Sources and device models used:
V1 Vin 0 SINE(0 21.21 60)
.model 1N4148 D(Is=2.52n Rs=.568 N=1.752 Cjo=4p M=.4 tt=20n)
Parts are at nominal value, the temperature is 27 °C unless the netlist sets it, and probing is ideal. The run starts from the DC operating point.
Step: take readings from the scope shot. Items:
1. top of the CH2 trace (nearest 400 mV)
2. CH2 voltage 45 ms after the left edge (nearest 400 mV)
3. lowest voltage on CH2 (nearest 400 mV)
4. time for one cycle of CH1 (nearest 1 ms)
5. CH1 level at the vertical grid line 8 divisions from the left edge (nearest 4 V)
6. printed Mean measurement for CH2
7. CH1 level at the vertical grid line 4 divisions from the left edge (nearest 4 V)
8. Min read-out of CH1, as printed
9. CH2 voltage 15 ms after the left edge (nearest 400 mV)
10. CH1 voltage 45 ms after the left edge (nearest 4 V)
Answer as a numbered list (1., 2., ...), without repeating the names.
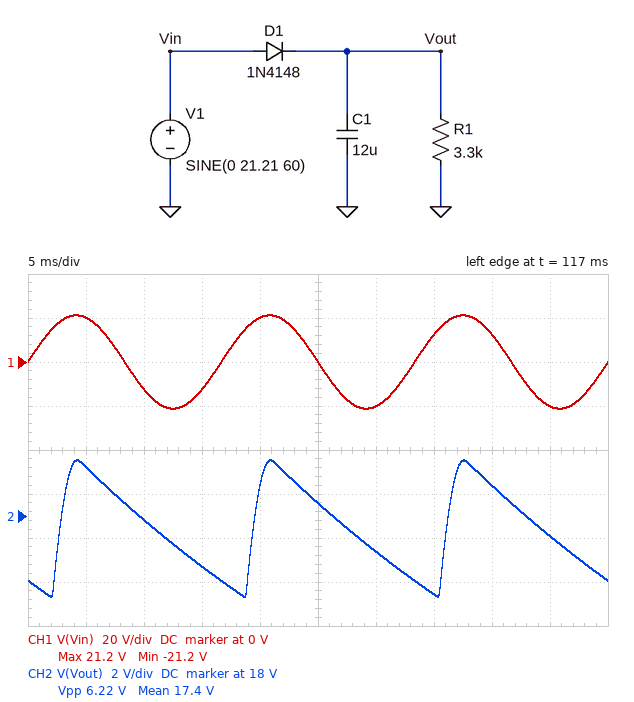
1. 20.4 V
2. 17.2 V
3. 14.4 V
4. 17 ms
5. 12 V
6. 17.4 V
7. 20 V
8. -21.2 V
9. 15.6 V
10. -20 V
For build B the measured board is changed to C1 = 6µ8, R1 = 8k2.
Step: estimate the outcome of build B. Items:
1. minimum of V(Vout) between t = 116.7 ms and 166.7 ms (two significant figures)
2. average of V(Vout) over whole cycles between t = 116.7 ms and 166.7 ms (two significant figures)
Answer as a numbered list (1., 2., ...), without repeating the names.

1. 16 V
2. 18 V
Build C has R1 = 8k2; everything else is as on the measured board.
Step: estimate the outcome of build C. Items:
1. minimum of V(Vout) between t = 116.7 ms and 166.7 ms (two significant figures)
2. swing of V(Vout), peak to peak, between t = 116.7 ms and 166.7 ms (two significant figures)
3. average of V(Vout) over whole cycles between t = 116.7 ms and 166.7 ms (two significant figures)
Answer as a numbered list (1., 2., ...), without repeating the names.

1. 18 V
2. 2.9 V
3. 19 V
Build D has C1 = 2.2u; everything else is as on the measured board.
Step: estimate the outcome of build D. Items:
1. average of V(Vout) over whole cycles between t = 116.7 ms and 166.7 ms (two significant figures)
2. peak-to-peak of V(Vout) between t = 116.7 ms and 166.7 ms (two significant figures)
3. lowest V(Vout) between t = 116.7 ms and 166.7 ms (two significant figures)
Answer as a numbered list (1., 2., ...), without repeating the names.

1. 11 V
2. 17 V
3. 3.7 V
